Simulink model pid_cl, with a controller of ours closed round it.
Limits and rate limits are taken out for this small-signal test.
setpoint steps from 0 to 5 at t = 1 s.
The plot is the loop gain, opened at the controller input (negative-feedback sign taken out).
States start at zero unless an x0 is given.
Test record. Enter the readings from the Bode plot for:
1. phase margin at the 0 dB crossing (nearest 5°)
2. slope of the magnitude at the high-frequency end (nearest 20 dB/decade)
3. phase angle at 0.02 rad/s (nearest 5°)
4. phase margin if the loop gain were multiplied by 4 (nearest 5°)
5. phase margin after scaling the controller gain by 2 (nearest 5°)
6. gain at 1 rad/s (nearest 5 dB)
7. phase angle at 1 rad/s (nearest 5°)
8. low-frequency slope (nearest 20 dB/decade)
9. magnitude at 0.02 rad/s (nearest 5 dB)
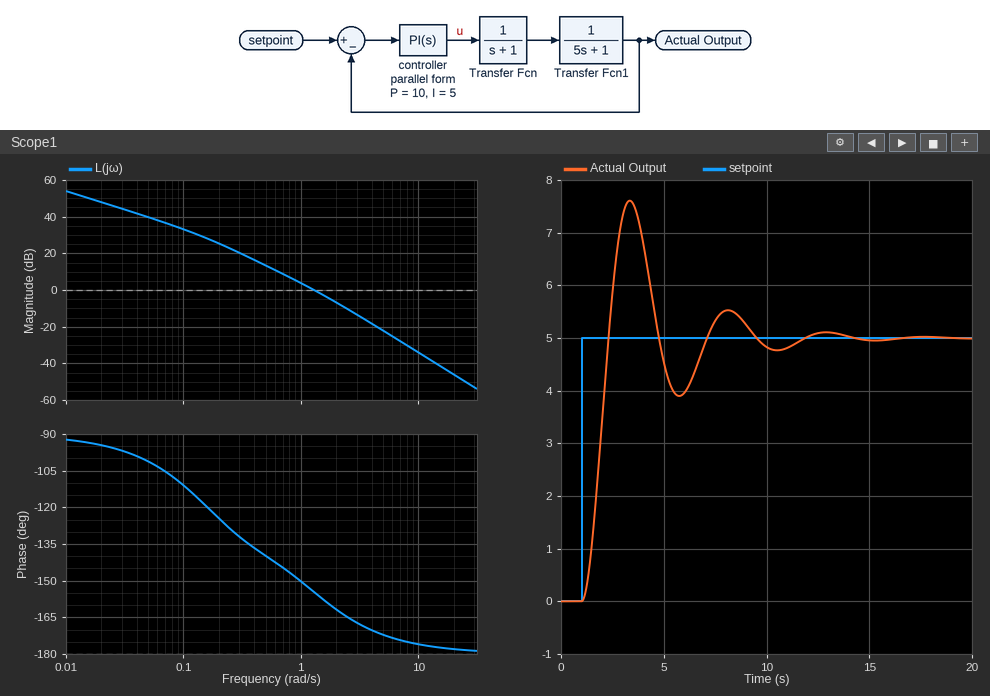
25°
-40 dB/decade
-95°
15°
20°
5 dB
-150°
-20 dB/decade
50 dB
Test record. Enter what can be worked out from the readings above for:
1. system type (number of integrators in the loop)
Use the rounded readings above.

1
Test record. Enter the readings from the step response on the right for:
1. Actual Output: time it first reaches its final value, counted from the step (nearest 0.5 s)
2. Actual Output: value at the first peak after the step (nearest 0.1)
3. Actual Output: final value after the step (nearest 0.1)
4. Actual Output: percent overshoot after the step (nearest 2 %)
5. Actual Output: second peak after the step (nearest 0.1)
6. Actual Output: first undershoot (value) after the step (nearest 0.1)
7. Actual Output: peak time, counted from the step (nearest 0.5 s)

1.5 s
7.6
5.0
52 %
5.5
3.9
2.5 s
